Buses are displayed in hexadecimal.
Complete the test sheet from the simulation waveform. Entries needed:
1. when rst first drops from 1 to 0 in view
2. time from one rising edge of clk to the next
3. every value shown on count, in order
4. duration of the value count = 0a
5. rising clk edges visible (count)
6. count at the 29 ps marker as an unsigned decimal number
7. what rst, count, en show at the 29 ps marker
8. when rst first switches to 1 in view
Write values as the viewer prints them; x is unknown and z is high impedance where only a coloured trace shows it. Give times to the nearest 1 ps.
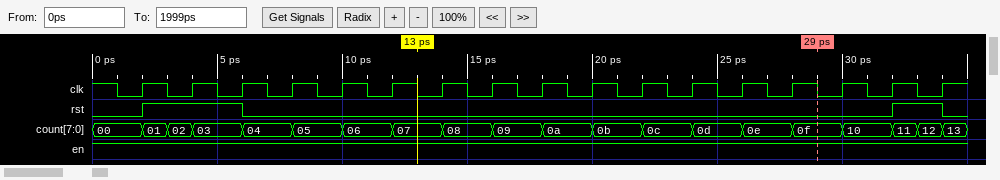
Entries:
6 ps
2 ps
00, 01, 02, 03, 04, 05, 06, 07, 08, 09, 0a, 0b, 0c, 0d, 0e, 0f, 10, 11, 12, 13
2 ps
17
15
rst=0, count=0f, en=1
2 ps
